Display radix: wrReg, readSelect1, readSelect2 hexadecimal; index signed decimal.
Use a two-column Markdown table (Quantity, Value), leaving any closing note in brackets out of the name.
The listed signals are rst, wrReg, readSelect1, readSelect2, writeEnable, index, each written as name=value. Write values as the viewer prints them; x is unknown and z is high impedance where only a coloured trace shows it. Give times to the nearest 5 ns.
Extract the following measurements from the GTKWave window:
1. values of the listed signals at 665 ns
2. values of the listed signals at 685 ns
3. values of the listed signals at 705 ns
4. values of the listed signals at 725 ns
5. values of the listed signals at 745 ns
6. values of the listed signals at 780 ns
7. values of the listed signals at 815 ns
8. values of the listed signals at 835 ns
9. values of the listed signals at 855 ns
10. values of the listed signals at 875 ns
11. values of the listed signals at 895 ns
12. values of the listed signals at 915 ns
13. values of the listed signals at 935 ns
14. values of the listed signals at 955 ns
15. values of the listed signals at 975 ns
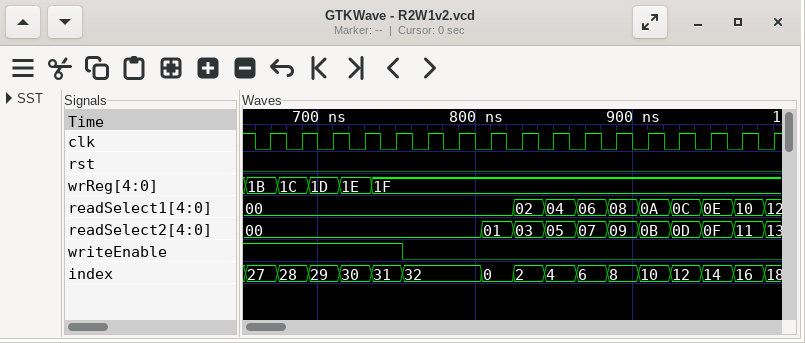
| Quantity | Value |
|---|---|
| values of the listed signals at 665 ns | rst=0, wrReg=1B, readSelect1=00, readSelect2=00, writeEnable=1, index=27 |
| values of the listed signals at 685 ns | rst=0, wrReg=1C, readSelect1=00, readSelect2=00, writeEnable=1, index=28 |
| values of the listed signals at 705 ns | rst=0, wrReg=1D, readSelect1=00, readSelect2=00, writeEnable=1, index=29 |
| values of the listed signals at 725 ns | rst=0, wrReg=1E, readSelect1=00, readSelect2=00, writeEnable=1, index=30 |
| values of the listed signals at 745 ns | rst=0, wrReg=1F, readSelect1=00, readSelect2=00, writeEnable=1, index=31 |
| values of the listed signals at 780 ns | rst=0, wrReg=1F, readSelect1=00, readSelect2=00, writeEnable=0, index=32 |
| values of the listed signals at 815 ns | rst=0, wrReg=1F, readSelect1=00, readSelect2=01, writeEnable=0, index=0 |
| values of the listed signals at 835 ns | rst=0, wrReg=1F, readSelect1=02, readSelect2=03, writeEnable=0, index=2 |
| values of the listed signals at 855 ns | rst=0, wrReg=1F, readSelect1=04, readSelect2=05, writeEnable=0, index=4 |
| values of the listed signals at 875 ns | rst=0, wrReg=1F, readSelect1=06, readSelect2=07, writeEnable=0, index=6 |
| values of the listed signals at 895 ns | rst=0, wrReg=1F, readSelect1=08, readSelect2=09, writeEnable=0, index=8 |
| values of the listed signals at 915 ns | rst=0, wrReg=1F, readSelect1=0A, readSelect2=0B, writeEnable=0, index=10 |
| values of the listed signals at 935 ns | rst=0, wrReg=1F, readSelect1=0C, readSelect2=0D, writeEnable=0, index=12 |
| values of the listed signals at 955 ns | rst=0, wrReg=1F, readSelect1=0E, readSelect2=0F, writeEnable=0, index=14 |
| values of the listed signals at 975 ns | rst=0, wrReg=1F, readSelect1=10, readSelect2=11, writeEnable=0, index=16 |
